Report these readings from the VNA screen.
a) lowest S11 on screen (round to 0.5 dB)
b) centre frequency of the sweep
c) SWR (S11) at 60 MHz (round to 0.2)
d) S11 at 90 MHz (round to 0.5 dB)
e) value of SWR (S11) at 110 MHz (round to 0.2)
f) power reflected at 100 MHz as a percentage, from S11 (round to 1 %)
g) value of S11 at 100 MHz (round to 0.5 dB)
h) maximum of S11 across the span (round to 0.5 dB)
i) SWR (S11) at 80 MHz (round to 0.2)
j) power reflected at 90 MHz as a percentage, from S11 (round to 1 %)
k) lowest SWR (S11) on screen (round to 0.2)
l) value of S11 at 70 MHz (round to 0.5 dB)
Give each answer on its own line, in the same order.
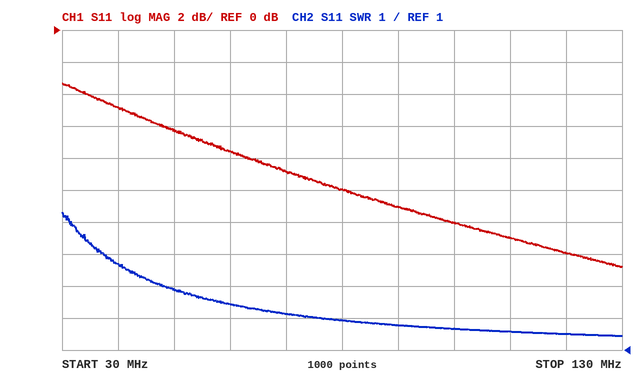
-15.0 dB
80 MHz
2.4
-11.0 dB
1.6
6 %
-12.0 dB
-3.5 dB
2.0
8 %
1.4
-9.0 dB
